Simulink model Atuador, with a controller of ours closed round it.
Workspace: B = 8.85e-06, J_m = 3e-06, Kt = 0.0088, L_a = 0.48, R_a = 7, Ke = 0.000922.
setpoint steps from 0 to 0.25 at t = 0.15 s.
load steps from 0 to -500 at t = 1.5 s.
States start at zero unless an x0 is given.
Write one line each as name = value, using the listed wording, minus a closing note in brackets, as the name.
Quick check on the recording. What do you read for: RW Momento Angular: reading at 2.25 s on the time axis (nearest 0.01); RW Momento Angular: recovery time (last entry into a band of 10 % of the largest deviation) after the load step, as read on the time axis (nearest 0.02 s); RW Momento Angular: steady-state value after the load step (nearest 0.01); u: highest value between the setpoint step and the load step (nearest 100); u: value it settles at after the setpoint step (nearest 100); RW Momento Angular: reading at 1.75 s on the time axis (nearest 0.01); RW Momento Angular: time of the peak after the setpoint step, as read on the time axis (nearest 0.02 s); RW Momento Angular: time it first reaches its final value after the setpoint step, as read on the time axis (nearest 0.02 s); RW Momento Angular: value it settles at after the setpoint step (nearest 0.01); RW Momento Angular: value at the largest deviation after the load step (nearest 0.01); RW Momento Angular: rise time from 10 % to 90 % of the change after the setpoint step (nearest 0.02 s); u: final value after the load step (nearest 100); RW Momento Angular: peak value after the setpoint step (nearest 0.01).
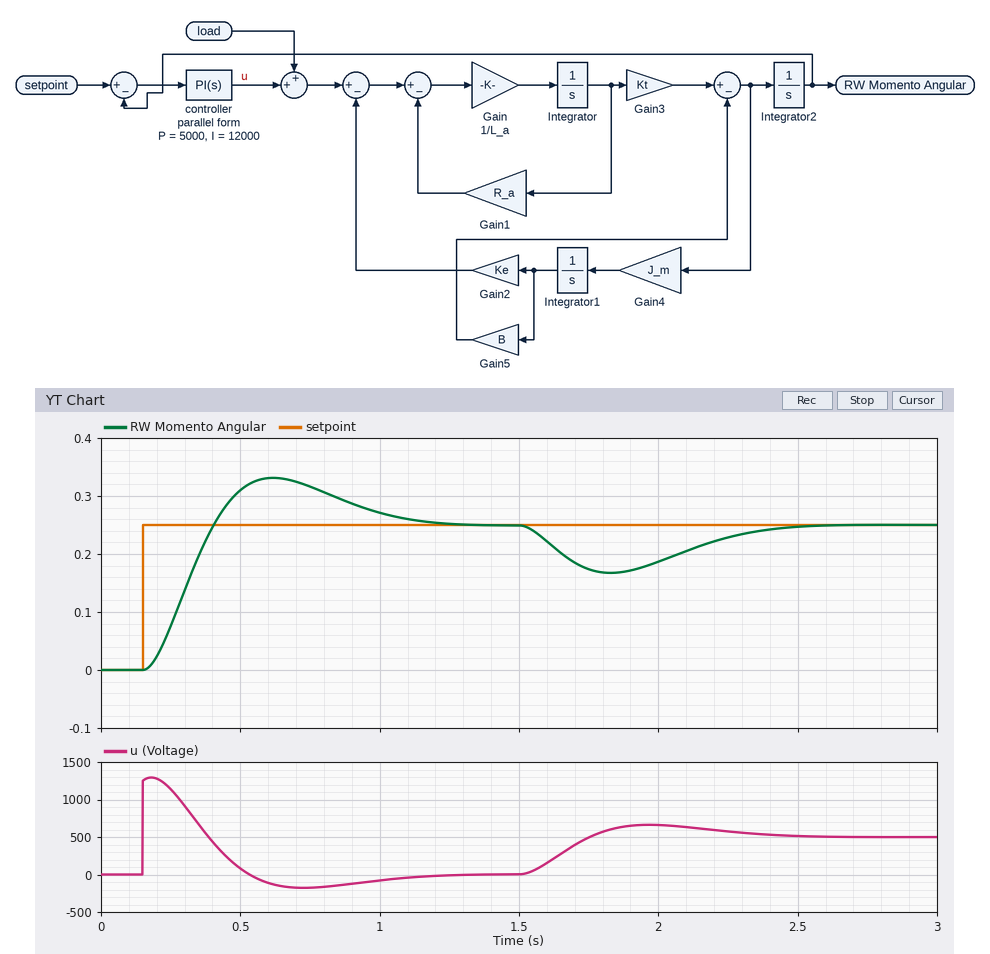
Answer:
RW Momento Angular: reading at 2.25 s on the time axis = 0.23
RW Momento Angular: recovery time (last entry into a band of 10 % of the largest deviation) after the load step, as read on the time axis = 2.40 s
RW Momento Angular: steady-state value after the load step = 0.25
u: highest value between the setpoint step and the load step = 1300
u: value it settles at after the setpoint step = 0
RW Momento Angular: reading at 1.75 s on the time axis = 0.17
RW Momento Angular: time of the peak after the setpoint step, as read on the time axis = 0.62 s
RW Momento Angular: time it first reaches its final value after the setpoint step, as read on the time axis = 0.40 s
RW Momento Angular: value it settles at after the setpoint step = 0.25
RW Momento Angular: value at the largest deviation after the load step = 0.17
RW Momento Angular: rise time from 10 % to 90 % of the change after the setpoint step = 0.18 s
u: final value after the load step = 500
RW Momento Angular: peak value after the setpoint step = 0.33
